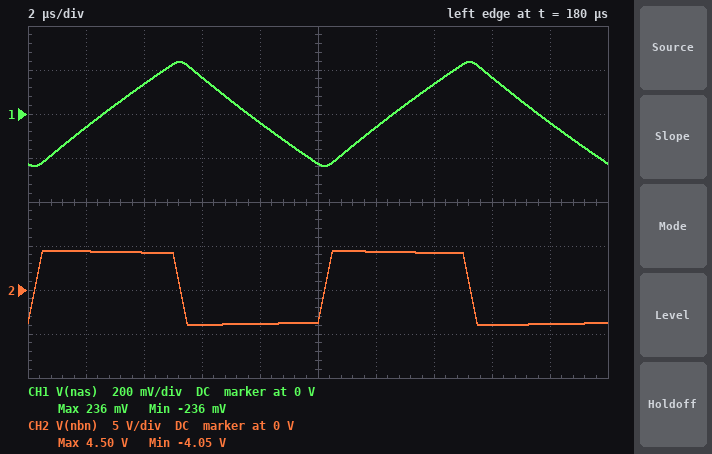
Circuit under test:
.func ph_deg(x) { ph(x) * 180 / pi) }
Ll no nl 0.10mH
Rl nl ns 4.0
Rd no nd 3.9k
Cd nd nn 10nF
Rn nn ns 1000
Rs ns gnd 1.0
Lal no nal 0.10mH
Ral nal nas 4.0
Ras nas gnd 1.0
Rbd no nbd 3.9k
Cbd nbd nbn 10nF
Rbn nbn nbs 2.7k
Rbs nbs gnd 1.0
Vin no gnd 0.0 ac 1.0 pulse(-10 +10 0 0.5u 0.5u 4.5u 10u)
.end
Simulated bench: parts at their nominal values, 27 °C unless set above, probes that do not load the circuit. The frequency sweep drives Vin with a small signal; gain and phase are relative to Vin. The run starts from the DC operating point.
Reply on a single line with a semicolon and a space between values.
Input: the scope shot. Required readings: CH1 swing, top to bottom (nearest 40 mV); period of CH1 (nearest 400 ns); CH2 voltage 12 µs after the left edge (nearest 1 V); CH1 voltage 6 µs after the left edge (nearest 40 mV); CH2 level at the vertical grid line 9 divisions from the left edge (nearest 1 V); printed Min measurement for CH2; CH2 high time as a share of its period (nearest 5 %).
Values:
480 mV; 10.0 µs; 4 V; 160 mV; -4 V; -4.05 V; 50 %
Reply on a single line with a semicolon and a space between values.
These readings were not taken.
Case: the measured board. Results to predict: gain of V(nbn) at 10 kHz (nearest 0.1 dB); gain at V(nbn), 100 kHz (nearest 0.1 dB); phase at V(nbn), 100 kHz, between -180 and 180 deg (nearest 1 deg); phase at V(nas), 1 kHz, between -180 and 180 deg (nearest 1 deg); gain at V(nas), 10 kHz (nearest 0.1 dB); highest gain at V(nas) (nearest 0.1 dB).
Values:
-8.0 dB; -7.8 dB; 1 deg; -7 deg; -18.1 dB; -14.0 dB
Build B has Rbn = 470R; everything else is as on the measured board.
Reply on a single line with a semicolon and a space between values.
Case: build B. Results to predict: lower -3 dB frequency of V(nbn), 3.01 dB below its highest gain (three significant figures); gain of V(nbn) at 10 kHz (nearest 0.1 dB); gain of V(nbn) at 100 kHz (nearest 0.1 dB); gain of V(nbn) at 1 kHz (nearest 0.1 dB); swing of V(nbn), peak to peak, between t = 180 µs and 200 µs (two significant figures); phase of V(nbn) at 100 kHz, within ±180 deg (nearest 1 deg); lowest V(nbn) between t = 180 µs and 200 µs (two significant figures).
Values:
3.64 kHz; -19.9 dB; -19.4 dB; -30.9 dB; 2.3 V; 2 deg; -1.1 V
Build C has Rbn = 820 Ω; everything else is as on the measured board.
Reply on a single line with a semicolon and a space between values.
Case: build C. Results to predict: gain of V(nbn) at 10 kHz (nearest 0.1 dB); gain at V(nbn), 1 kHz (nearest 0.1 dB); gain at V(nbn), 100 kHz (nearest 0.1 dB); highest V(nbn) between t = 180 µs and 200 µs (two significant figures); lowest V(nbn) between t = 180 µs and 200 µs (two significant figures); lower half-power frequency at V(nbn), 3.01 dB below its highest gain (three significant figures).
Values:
-15.7 dB; -26.1 dB; -15.2 dB; 1.9 V; -1.8 V; 3.37 kHz
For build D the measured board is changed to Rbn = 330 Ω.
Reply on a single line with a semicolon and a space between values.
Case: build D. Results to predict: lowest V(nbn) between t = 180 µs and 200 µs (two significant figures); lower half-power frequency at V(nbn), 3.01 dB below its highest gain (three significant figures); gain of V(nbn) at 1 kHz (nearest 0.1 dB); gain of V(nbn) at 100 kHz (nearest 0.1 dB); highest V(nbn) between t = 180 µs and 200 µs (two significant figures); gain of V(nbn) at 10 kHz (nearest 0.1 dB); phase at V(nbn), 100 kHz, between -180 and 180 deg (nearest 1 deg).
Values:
-820 mV; 3.76 kHz; -33.9 dB; -22.1 dB; 830 mV; -22.7 dB; 2 deg
